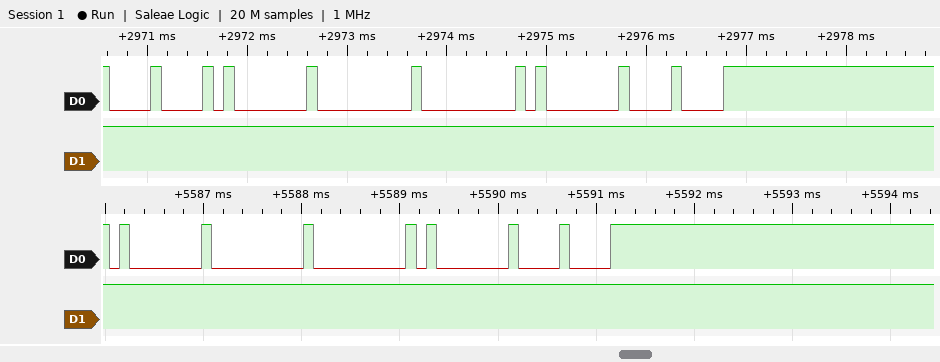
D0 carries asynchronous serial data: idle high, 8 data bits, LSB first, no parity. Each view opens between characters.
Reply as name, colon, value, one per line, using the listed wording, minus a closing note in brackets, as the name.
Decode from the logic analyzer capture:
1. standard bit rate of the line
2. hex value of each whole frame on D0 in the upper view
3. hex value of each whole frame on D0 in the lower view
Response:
standard bit rate of the line: 9600 baud
hex value of each whole frame on D0 in the upper view: 08, 01, 00, 00, 01, 08
hex value of each whole frame on D0 in the lower view: 01, 00, 00, 01, 08
